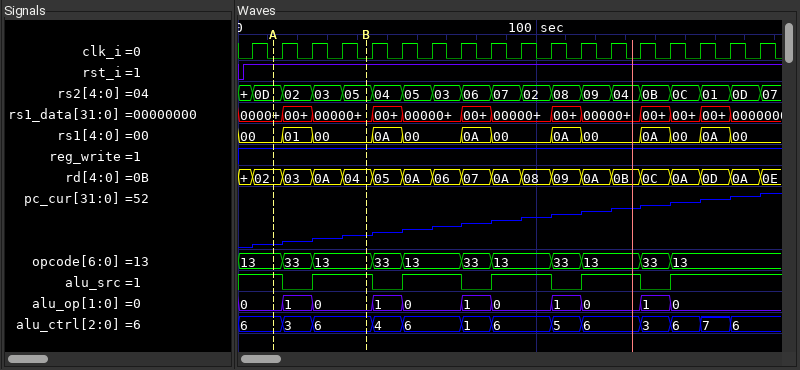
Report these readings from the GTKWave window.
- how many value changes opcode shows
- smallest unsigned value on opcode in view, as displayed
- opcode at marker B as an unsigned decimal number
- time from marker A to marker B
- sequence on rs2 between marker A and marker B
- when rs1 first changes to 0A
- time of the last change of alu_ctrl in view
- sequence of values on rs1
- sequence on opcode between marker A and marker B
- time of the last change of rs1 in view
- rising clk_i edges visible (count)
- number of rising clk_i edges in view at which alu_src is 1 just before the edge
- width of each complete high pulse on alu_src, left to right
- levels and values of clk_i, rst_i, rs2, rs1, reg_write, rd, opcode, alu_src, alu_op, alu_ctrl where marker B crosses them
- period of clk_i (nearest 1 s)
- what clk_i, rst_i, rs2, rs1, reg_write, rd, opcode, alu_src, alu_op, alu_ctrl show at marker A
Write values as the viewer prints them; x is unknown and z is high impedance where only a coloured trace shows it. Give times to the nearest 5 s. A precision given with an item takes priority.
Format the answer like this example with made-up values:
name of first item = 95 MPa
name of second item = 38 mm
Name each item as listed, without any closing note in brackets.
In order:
how many value changes opcode shows = 10
smallest unsigned value on opcode in view, as displayed = 13
opcode at marker B as an unsigned decimal number = 19
time from marker A to marker B = 30 s
sequence on rs2 between marker A and marker B = 0D, 02, 03, 05
when rs1 first changes to 0A = 45 s
time of the last change of alu_ctrl in view = 165 s
sequence of values on rs1 = 00, 01, 00, 0A, 00, 0A, 00, 0A, 00, 0A, 00, 0A, 00
sequence on opcode between marker A and marker B = 13, 33, 13
time of the last change of rs1 in view = 165 s
rising clk_i edges visible = 18
number of rising clk_i edges in view at which alu_src is 1 just before the edge = 13
width of each complete high pulse on alu_src, left to right = 20 s, 20 s, 20 s, 20 s
levels and values of clk_i, rst_i, rs2, rs1, reg_write, rd, opcode, alu_src, alu_op, alu_ctrl where marker B crosses them = clk_i=0, rst_i=1, rs2=05, rs1=00, reg_write=1, rd=04, opcode=13, alu_src=1, alu_op=0, alu_ctrl=6
period of clk_i = 10 s
what clk_i, rst_i, rs2, rs1, reg_write, rd, opcode, alu_src, alu_op, alu_ctrl show at marker A = clk_i=0, rst_i=1, rs2=0D, rs1=00, reg_write=1, rd=02, opcode=13, alu_src=1, alu_op=0, alu_ctrl=6
